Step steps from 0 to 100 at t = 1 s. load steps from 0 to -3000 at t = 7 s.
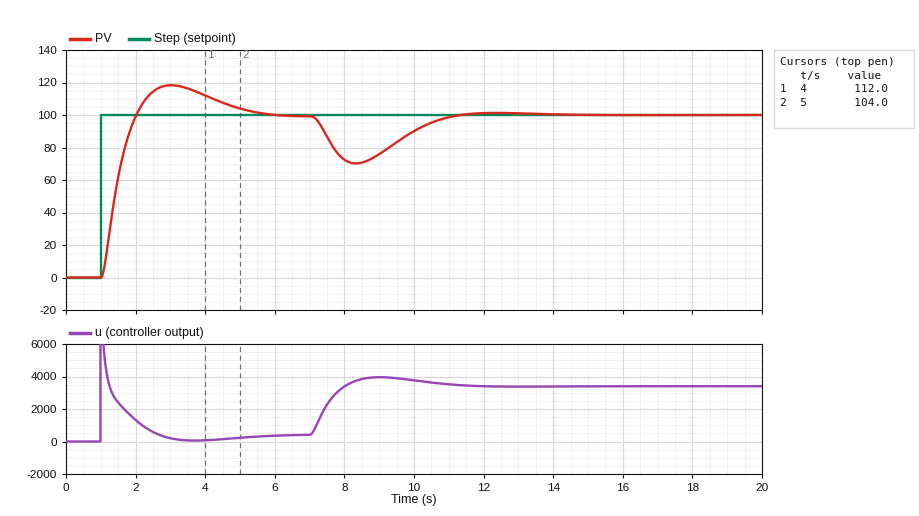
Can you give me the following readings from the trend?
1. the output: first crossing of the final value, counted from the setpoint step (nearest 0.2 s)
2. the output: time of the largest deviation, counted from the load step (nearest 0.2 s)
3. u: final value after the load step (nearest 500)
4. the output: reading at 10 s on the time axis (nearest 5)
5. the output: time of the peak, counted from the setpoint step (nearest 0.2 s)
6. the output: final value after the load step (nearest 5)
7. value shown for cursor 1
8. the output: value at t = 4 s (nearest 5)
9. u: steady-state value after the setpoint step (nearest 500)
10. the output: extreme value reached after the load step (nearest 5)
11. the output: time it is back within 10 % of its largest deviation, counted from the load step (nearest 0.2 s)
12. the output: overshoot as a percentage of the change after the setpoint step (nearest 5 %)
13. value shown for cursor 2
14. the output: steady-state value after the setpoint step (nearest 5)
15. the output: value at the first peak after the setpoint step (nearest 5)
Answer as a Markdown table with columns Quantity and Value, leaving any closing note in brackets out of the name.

| Quantity | Value |
|---|---|
| the output: first crossing of the final value, counted from the setpoint step | 1.0 s |
| the output: time of the largest deviation, counted from the load step | 1.4 s |
| u: final value after the load step | 3500 |
| the output: reading at 10 s on the time axis | 90 |
| the output: time of the peak, counted from the setpoint step | 2.0 s |
| the output: final value after the load step | 100 |
| value shown for cursor 1 | 112.0 |
| the output: value at t = 4 s | 110 |
| u: steady-state value after the setpoint step | 500 |
| the output: extreme value reached after the load step | 70 |
| the output: time it is back within 10 % of its largest deviation, counted from the load step | 3.8 s |
| the output: overshoot as a percentage of the change after the setpoint step | 20 % |
| value shown for cursor 2 | 104.0 |
| the output: steady-state value after the setpoint step | 100 |
| the output: value at the first peak after the setpoint step | 120 |
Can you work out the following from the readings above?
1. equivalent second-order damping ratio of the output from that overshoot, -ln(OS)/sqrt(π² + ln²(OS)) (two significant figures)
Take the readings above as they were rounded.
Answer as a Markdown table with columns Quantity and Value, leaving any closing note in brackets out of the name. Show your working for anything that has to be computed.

| Quantity | Value |
|---|---|
| equivalent second-order damping ratio of the output from that overshoot, -ln(OS)/sqrt(π² + ln²(OS)) | ln(0.2) = -1.609; 1.609 / sqrt(9.870 + 2.590) = 0.46 |
